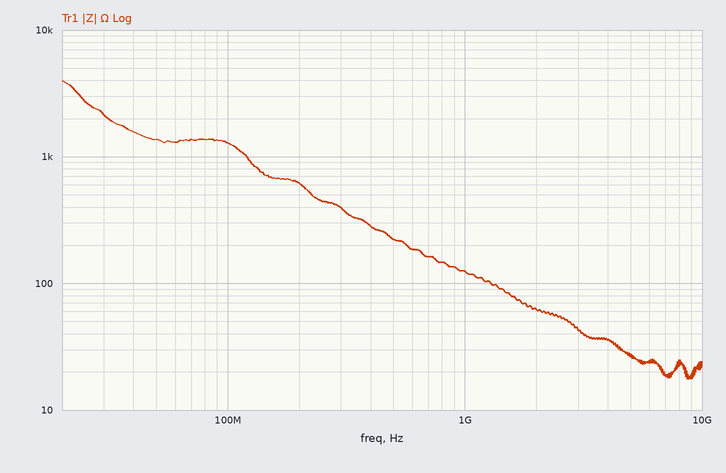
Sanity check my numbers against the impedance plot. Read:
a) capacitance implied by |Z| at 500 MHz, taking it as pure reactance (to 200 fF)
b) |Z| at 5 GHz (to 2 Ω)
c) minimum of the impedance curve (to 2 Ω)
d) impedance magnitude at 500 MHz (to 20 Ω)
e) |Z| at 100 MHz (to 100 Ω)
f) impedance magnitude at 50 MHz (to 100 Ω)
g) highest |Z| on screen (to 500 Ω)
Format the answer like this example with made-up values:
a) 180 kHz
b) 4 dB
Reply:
a) 1.4 pF
b) 26 Ω
c) 18 Ω
d) 220 Ω
e) 1.3 kΩ
f) 1.4 kΩ
g) 4.0 kΩ
